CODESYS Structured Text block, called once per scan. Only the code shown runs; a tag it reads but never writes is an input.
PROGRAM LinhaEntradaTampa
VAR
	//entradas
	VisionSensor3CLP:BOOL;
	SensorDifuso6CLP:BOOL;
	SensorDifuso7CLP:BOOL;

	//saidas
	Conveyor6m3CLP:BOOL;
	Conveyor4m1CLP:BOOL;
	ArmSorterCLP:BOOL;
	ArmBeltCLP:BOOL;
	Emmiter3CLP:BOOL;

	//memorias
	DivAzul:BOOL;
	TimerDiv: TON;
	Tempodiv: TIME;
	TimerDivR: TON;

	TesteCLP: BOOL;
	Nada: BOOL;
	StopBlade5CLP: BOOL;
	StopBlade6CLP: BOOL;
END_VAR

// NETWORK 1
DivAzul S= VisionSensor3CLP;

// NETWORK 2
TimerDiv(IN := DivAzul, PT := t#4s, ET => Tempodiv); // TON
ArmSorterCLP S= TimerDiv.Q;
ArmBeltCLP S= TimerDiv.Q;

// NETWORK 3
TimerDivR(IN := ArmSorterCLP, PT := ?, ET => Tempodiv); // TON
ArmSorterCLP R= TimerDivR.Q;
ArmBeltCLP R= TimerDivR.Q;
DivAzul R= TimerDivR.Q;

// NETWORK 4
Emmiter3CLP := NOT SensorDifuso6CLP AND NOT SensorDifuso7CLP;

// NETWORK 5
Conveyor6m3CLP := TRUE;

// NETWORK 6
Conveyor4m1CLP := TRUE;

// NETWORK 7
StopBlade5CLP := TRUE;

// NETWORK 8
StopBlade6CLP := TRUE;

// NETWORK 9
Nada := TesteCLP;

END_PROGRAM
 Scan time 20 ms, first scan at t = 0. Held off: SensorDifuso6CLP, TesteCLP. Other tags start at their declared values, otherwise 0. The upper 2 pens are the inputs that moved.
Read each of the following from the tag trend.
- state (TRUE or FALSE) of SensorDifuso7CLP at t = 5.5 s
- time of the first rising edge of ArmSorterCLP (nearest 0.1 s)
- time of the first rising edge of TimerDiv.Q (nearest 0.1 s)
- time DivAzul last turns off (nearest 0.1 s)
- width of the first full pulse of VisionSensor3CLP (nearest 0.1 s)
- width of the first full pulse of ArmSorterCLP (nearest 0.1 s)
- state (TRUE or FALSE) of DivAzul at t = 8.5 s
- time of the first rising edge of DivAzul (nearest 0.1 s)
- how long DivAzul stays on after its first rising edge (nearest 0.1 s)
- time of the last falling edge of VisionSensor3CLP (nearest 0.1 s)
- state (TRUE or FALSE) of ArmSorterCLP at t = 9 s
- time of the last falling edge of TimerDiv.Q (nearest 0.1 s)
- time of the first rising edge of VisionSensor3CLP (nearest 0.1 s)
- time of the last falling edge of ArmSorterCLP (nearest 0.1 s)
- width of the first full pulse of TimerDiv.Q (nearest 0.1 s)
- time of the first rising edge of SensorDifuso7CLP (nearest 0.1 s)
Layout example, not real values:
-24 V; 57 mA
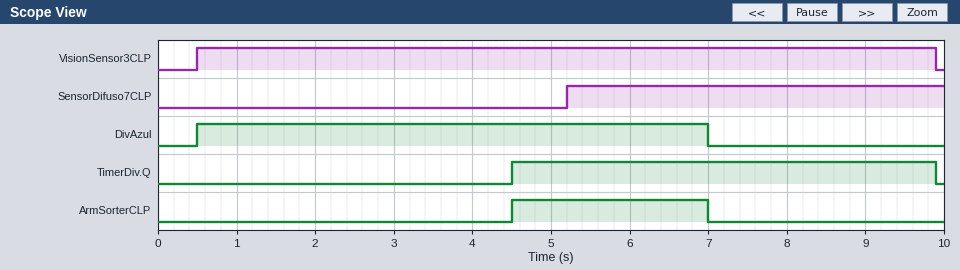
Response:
TRUE; 4.5 s; 4.5 s; 7.0 s; 9.4 s; 2.5 s; FALSE; 0.5 s; 6.5 s; 9.9 s; FALSE; 9.9 s; 0.5 s; 7.0 s; 5.4 s; 5.2 s
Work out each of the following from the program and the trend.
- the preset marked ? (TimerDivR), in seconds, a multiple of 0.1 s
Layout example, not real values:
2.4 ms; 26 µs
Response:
2.5 s
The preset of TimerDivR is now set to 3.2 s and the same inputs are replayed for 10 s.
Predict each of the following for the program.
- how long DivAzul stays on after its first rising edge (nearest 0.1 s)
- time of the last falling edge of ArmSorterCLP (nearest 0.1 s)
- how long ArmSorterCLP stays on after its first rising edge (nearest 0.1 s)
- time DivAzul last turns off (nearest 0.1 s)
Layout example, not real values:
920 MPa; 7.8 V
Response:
7.2 s; 7.7 s; 3.2 s; 7.7 s
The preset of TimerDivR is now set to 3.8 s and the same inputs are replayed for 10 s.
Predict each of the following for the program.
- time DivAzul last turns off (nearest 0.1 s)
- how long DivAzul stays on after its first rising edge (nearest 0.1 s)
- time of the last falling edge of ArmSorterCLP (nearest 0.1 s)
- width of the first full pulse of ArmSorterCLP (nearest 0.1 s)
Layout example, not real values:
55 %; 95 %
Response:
8.3 s; 7.8 s; 8.3 s; 3.8 s
